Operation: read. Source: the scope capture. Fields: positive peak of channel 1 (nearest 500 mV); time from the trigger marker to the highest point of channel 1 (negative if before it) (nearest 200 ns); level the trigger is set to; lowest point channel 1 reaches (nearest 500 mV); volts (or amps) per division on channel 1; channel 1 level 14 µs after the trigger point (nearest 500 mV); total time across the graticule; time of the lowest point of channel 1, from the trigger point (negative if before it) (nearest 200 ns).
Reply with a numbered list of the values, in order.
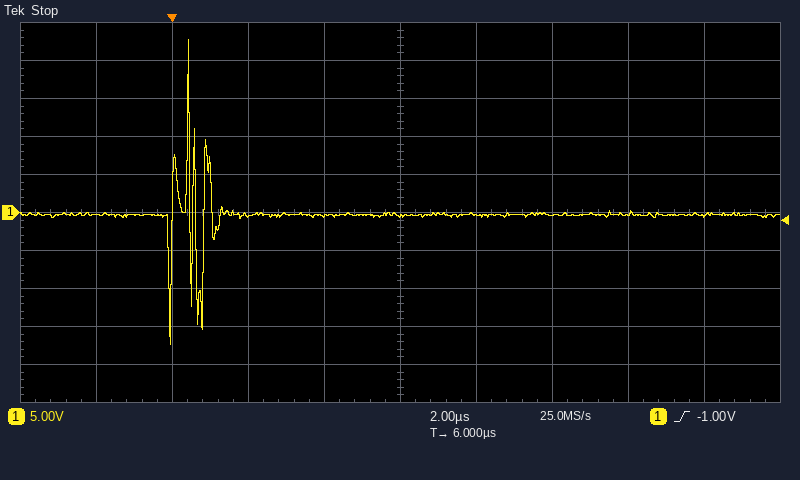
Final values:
1. 23.0 V
2. +400 ns
3. -1.00 V
4. -17.5 V
5. 5 V
6. -500 mV
7. 20 µs
8. 0.0 µs
